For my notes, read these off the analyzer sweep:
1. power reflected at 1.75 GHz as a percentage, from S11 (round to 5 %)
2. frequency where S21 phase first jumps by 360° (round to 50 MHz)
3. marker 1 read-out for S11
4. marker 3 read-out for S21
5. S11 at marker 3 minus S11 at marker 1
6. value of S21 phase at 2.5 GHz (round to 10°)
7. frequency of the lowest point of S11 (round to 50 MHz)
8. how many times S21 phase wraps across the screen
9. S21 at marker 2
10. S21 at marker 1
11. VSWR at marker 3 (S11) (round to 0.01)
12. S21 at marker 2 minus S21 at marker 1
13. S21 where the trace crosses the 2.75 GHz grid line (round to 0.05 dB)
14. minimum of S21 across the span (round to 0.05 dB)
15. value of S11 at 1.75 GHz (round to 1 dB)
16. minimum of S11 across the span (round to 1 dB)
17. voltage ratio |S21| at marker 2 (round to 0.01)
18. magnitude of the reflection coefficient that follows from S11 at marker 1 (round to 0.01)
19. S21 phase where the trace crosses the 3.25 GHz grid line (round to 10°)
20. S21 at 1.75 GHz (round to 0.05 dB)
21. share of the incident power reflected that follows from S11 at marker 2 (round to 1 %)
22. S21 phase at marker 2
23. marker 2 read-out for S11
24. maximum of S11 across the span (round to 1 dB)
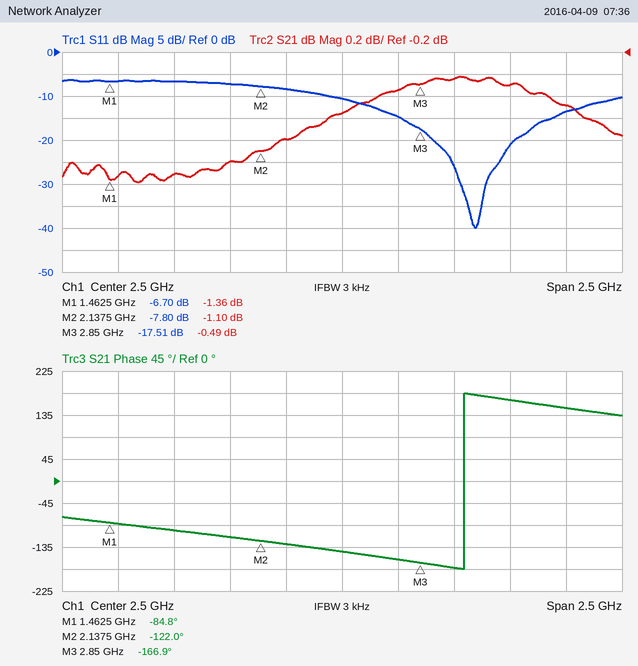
20 %
3.05 GHz
-6.70 dB
-0.49 dB
-10.81 dB
-140°
3.10 GHz
1
-1.10 dB
-1.36 dB
1.31
0.26 dB
-0.55 dB
-1.40 dB
-7 dB
-40 dB
0.88
0.46
170°
-1.30 dB
17 %
-122.0°
-7.80 dB
-6 dB
